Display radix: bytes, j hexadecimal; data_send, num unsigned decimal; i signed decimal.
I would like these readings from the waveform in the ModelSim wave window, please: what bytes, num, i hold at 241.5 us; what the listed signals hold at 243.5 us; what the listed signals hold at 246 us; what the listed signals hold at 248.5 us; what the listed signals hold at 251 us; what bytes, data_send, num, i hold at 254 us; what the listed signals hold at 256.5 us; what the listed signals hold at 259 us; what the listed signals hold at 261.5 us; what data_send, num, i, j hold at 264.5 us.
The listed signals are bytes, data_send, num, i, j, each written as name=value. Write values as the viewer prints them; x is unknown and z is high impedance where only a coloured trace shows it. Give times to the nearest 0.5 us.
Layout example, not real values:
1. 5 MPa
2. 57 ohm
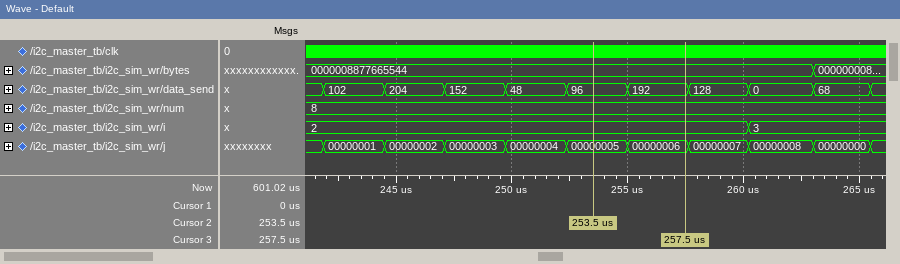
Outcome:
1. bytes=0000008877665544, num=8, i=2
2. bytes=0000008877665544, data_send=102, num=8, i=2, j=00000001
3. bytes=0000008877665544, data_send=204, num=8, i=2, j=00000002
4. bytes=0000008877665544, data_send=152, num=8, i=2, j=00000003
5. bytes=0000008877665544, data_send=48, num=8, i=2, j=00000004
6. bytes=0000008877665544, data_send=96, num=8, i=2
7. bytes=0000008877665544, data_send=192, num=8, i=2, j=00000006
8. bytes=0000008877665544, data_send=128, num=8, i=2, j=00000007
9. bytes=0000008877665544, data_send=0, num=8, i=3, j=00000008
10. data_send=68, num=8, i=3, j=00000000
